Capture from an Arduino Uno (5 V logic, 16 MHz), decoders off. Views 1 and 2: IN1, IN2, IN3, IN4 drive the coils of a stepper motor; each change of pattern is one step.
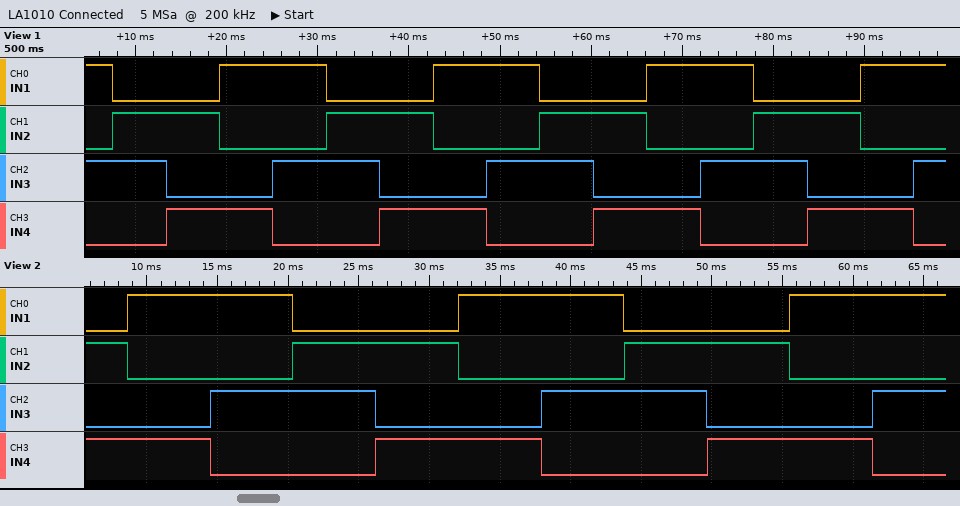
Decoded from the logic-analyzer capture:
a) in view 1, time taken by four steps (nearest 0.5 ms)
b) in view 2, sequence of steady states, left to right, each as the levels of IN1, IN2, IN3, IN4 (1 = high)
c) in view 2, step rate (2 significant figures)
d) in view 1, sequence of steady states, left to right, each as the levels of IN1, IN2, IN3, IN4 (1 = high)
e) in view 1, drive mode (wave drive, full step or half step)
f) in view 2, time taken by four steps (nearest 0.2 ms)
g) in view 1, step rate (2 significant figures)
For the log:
23.5 ms
0101 1001 1010 0110 0101 1001 1010 0110 0101 1001 1010
170 steps/s
1010 0110 0101 1001 1010 0110 0101 1001 1010 0110 0101 1001 1010 0110 0101 1001 1010
full step
23.4 ms
170 steps/s
